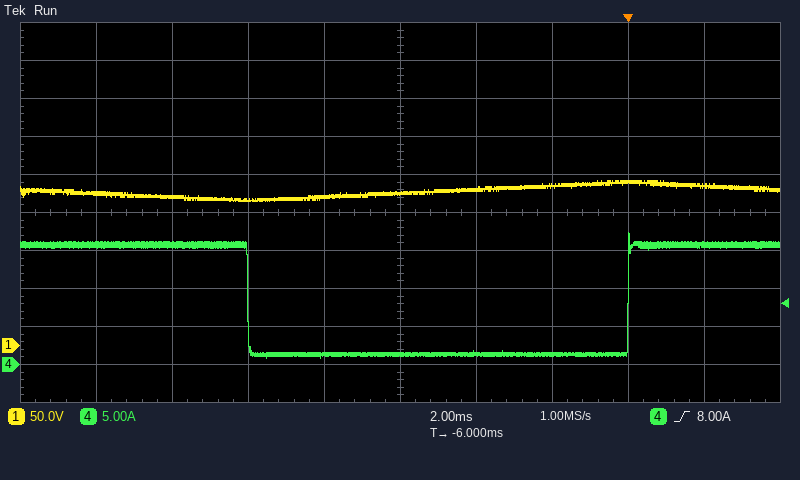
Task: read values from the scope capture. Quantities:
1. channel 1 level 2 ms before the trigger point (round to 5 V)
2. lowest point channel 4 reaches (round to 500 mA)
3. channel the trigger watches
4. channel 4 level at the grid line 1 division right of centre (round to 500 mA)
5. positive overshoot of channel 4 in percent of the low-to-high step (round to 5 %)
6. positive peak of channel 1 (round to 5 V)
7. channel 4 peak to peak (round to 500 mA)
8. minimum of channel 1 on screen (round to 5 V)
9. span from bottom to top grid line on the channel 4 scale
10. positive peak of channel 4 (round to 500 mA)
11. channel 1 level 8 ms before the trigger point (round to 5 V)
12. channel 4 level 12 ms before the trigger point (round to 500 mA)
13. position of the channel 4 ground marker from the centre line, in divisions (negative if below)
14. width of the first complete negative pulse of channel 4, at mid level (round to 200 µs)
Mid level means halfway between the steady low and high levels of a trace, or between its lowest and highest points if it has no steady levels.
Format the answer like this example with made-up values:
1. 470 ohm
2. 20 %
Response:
1. 210 V
2. 1.0 A
3. channel 4
4. 1.5 A
5. 10 %
6. 215 V
7. 16.5 A
8. 190 V
9. 50 A
10. 17.5 A
11. 195 V
12. 15.5 A
13. -4.0 div
14. 10.0 ms
